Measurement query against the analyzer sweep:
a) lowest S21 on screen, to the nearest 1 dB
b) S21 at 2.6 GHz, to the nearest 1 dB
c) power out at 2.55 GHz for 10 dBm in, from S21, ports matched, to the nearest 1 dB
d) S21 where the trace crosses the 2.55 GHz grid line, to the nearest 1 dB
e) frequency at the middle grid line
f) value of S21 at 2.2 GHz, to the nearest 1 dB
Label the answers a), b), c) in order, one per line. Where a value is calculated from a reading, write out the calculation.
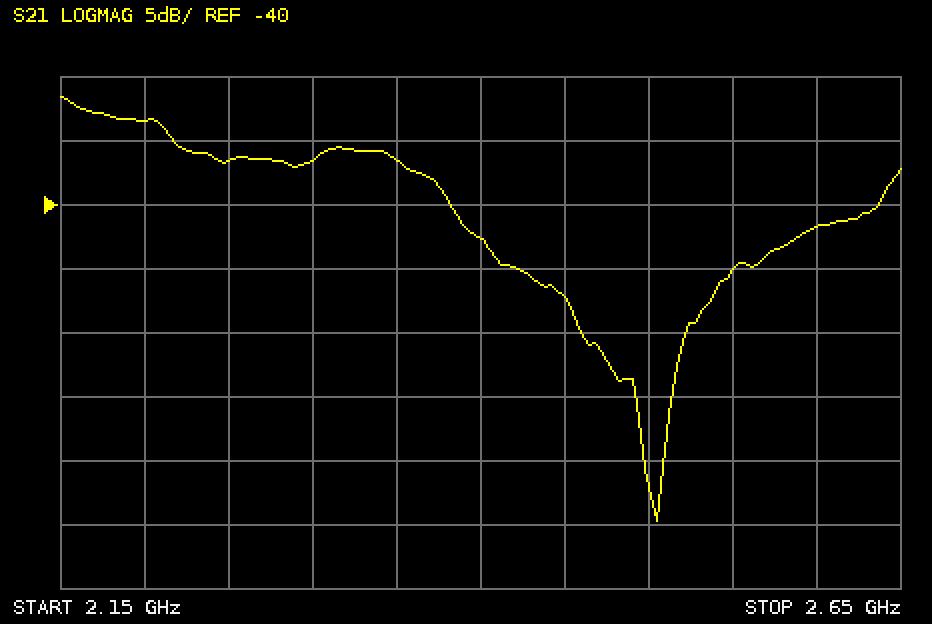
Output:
a) -65 dB
b) -42 dB
c) 10 dBm + (-45 dB) = -35 dBm
d) -45 dB
e) 2.4 GHz
f) -33 dB
